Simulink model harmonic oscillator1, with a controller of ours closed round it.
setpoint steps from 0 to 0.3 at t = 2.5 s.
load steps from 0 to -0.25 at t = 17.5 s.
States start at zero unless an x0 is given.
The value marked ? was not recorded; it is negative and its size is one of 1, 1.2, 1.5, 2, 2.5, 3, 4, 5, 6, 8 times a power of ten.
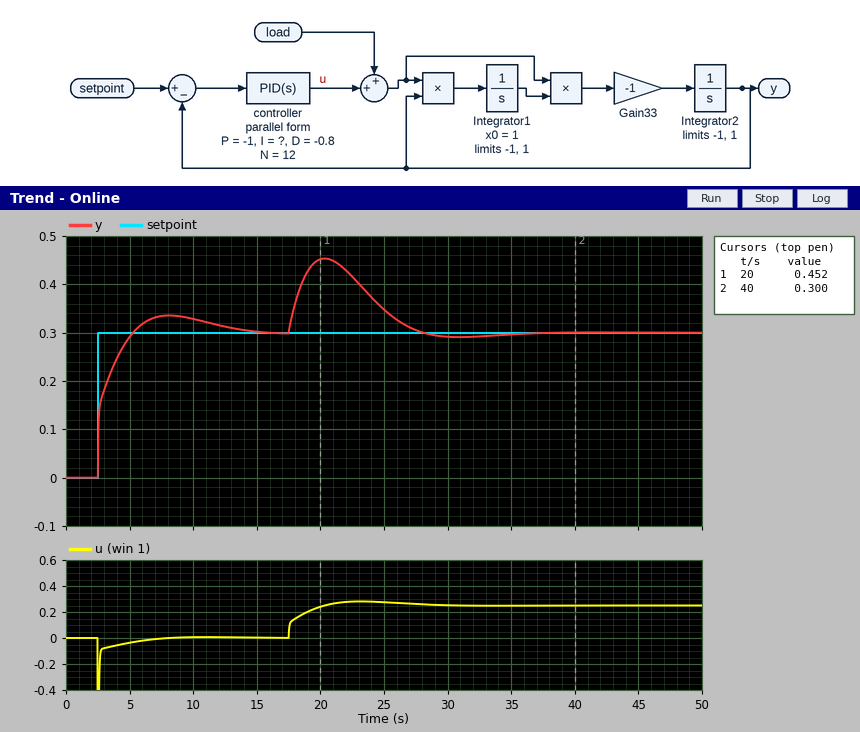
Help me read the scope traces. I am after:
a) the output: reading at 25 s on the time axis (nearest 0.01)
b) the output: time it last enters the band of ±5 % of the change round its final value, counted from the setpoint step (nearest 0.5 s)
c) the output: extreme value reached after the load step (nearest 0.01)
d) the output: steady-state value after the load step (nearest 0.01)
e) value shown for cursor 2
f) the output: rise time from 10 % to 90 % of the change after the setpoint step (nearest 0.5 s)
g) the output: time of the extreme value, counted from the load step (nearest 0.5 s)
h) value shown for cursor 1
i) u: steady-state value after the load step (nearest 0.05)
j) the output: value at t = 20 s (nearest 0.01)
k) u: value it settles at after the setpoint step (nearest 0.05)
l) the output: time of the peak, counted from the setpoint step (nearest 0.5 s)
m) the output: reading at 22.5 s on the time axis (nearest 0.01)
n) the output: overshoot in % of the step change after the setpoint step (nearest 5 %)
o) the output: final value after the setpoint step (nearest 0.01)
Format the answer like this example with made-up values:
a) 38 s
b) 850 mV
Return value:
a) 0.35
b) 9.5 s
c) 0.45
d) 0.30
e) 0.300
f) 2.0 s
g) 3.0 s
h) 0.452
i) 0.25
j) 0.45
k) 0.00
l) 5.5 s
m) 0.42
n) 10 %
o) 0.30
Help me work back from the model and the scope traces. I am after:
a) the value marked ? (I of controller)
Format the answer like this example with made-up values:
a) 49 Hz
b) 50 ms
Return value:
a) -0.3
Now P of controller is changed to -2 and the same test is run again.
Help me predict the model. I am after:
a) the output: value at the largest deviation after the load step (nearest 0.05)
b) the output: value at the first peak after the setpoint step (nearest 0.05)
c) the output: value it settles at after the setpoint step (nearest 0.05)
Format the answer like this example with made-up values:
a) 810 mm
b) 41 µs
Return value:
a) 0.40
b) 0.30
c) 0.30
